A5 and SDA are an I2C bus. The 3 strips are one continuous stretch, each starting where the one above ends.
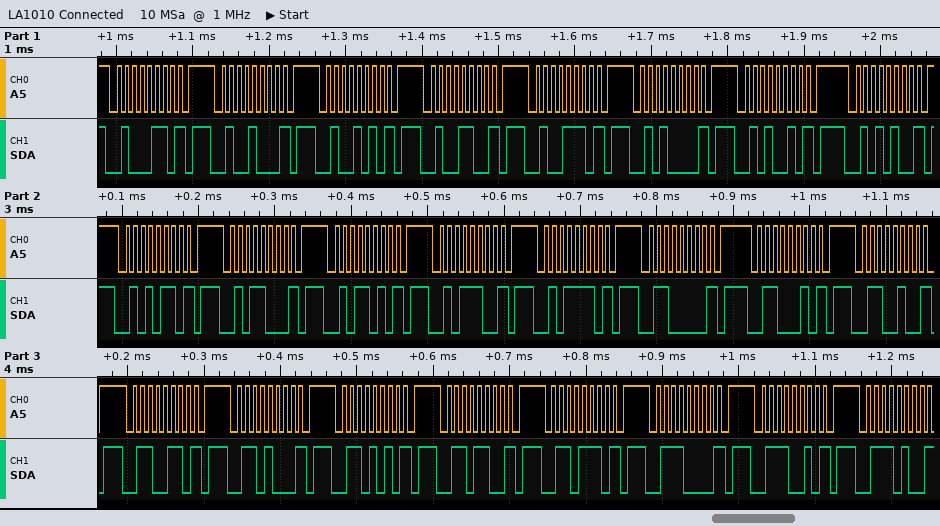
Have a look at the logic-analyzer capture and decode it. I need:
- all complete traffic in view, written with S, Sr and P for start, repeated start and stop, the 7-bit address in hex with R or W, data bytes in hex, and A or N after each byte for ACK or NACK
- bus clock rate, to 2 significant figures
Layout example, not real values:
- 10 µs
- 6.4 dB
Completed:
- S 23W N P S 24W N P S 25W N P S 26W N P S 27W N P S 28W N P S 29W N P S 2AW N P S 2BW N P S 2CW N P S 2DW N P S 2EW N P S 2FW N P S 30W N P S 31W N P S 32W N P S 33W N P S 34W N P S 35W N P S 36W N P S 37W N P S 38W N P S 39W N P S 3AW N
- 100 kHz
